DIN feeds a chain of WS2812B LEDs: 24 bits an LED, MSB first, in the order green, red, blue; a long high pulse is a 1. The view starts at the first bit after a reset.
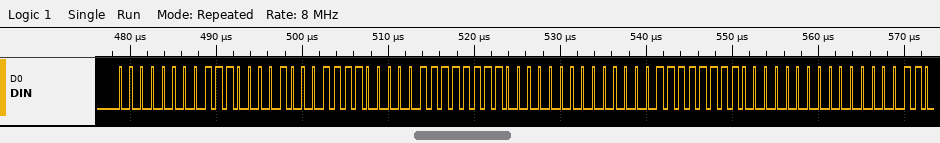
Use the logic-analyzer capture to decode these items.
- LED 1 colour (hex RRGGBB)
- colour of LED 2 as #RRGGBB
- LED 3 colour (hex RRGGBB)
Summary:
#E1001E
#F00F00
#C03F00
